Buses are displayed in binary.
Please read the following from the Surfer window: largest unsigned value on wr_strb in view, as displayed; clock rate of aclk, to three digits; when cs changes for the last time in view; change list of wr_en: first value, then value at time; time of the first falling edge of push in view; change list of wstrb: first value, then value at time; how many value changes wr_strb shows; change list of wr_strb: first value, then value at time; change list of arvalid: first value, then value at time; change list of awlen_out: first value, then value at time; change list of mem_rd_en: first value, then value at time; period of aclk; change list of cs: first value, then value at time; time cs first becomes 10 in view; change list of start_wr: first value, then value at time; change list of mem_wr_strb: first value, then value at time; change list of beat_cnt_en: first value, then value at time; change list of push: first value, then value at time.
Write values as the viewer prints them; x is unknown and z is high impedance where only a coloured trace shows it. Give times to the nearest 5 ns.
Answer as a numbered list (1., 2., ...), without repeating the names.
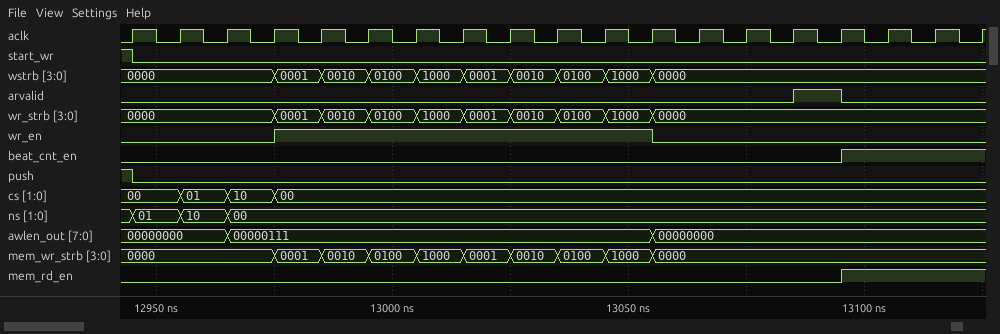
1. 1000
2. 100 MHz
3. 12975 ns
4. 0, 1 at 12975 ns, 0 at 13055 ns
5. 12945 ns
6. 0000, 0001 at 12975 ns, 0010 at 12985 ns, 0100 at 12995 ns, 1000 at 13005 ns, 0001 at 13015 ns, 0010 at 13025 ns, 0100 at 13035 ns, 1000 at 13045 ns, 0000 at 13055 ns
7. 9
8. 0000, 0001 at 12975 ns, 0010 at 12985 ns, 0100 at 12995 ns, 1000 at 13005 ns, 0001 at 13015 ns, 0010 at 13025 ns, 0100 at 13035 ns, 1000 at 13045 ns, 0000 at 13055 ns
9. 0, 1 at 13085 ns, 0 at 13095 ns
10. 00000000, 00000111 at 12965 ns, 00000000 at 13055 ns
11. 0, 1 at 13095 ns
12. 10 ns
13. 00, 01 at 12955 ns, 10 at 12965 ns, 00 at 12975 ns
14. 12965 ns
15. 1, 0 at 12945 ns
16. 0000, 0001 at 12975 ns, 0010 at 12985 ns, 0100 at 12995 ns, 1000 at 13005 ns, 0001 at 13015 ns, 0010 at 13025 ns, 0100 at 13035 ns, 1000 at 13045 ns, 0000 at 13055 ns
17. 0, 1 at 13095 ns
18. 1, 0 at 12945 ns
